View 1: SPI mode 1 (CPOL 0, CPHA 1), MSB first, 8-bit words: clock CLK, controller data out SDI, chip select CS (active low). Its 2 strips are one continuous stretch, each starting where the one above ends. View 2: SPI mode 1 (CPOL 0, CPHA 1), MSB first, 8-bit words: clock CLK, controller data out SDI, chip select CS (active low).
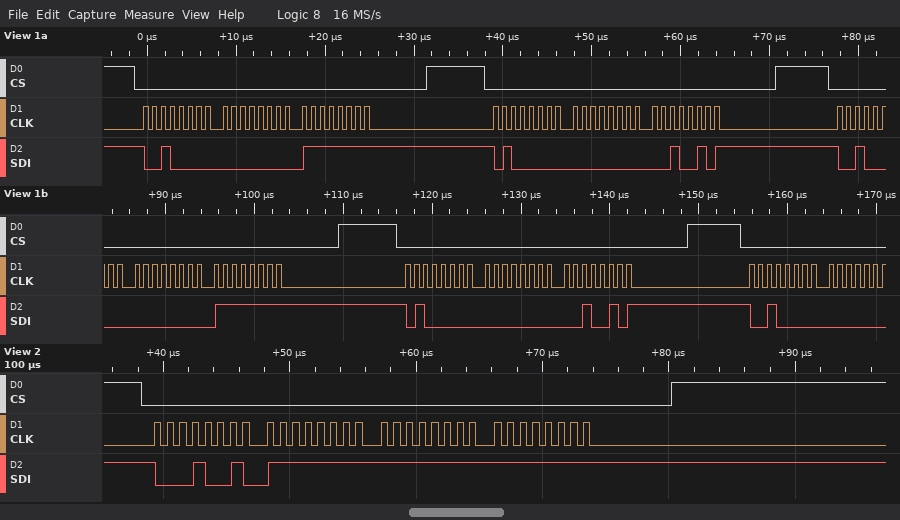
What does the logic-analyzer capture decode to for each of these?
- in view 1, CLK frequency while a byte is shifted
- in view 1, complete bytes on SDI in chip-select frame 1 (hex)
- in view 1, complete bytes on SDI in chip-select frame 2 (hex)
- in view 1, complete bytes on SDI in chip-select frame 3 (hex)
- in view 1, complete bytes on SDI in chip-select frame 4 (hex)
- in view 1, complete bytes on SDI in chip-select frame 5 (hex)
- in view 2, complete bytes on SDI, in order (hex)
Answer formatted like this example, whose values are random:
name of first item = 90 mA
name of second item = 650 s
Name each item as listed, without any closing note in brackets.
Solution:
in view 1, CLK frequency while a byte is shifted = 1 MHz
in view 1, complete bytes on SDI in chip-select frame 1 = 0x20 0x00 0xFF
in view 1, complete bytes on SDI in chip-select frame 2 = 0x40 0x00 0x25
in view 1, complete bytes on SDI in chip-select frame 3 = 0x20 0x00 0xFF
in view 1, complete bytes on SDI in chip-select frame 4 = 0x40 0x00 0x25
in view 1, complete bytes on SDI in chip-select frame 5 = 0x20
in view 2, complete bytes on SDI, in order = 12 FF FF FF
